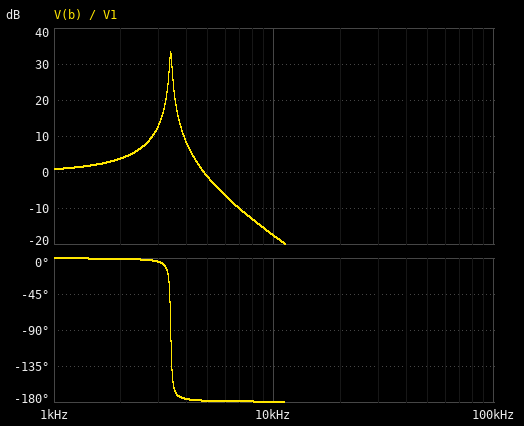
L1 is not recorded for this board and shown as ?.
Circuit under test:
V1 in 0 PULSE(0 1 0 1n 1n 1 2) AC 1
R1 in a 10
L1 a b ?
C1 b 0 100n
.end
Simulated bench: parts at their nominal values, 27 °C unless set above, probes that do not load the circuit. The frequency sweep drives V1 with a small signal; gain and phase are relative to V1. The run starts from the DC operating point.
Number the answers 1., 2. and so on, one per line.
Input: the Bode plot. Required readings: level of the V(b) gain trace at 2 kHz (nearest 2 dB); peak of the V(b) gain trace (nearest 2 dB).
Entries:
1. 4 dB
2. 34 dB
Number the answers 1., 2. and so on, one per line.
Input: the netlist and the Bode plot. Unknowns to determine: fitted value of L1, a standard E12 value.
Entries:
1. 22 mH
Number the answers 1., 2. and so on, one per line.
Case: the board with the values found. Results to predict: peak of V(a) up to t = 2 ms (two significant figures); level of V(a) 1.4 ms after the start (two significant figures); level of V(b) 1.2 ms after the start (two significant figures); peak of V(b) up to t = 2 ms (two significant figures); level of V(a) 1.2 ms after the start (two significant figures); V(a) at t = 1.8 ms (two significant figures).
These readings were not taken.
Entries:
1. 1.0 V
2. 1.0 V
3. 310 mV
4. 2.0 V
5. 990 mV
6. 990 mV
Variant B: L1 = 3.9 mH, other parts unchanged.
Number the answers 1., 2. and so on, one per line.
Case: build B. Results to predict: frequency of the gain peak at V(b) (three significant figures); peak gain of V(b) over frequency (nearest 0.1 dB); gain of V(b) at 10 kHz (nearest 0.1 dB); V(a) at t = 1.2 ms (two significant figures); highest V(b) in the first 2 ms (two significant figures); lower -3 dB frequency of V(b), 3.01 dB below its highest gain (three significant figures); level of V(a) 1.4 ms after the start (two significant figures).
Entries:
1. 8.05 kHz
2. 25.9 dB
3. 5.3 dB
4. 1.0 V
5. 1.9 V
6. 7.85 kHz
7. 990 mV
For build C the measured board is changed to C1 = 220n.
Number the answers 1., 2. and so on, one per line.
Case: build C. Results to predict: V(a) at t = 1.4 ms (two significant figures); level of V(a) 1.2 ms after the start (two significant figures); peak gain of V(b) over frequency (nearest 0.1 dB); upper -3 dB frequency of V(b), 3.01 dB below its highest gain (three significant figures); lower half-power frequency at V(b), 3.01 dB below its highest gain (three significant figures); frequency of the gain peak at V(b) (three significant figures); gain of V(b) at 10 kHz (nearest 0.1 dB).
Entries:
1. 980 mV
2. 1.0 V
3. 30.0 dB
4. 2.32 kHz
5. 2.25 kHz
6. 2.29 kHz
7. -25.2 dB
